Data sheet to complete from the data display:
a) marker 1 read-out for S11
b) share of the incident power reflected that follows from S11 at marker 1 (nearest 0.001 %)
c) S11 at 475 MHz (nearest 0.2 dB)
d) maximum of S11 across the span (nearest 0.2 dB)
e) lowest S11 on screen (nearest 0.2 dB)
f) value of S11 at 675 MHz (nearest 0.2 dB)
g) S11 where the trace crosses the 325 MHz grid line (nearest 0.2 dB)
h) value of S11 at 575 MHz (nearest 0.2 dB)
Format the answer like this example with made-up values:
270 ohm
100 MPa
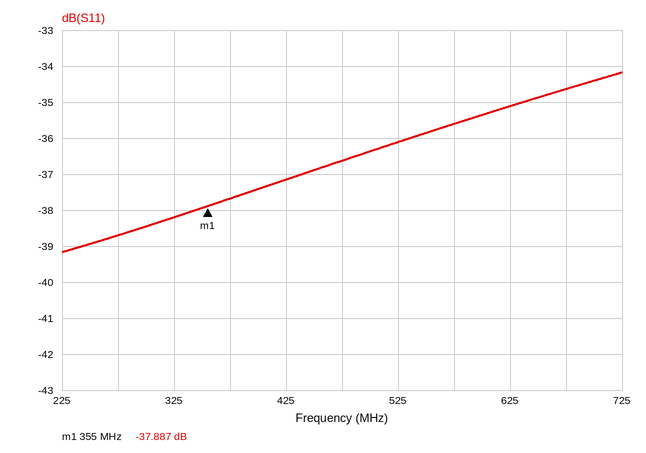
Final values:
-37.887 dB
0.016 %
-36.6 dB
-34.2 dB
-39.2 dB
-34.6 dB
-38.2 dB
-35.6 dB
